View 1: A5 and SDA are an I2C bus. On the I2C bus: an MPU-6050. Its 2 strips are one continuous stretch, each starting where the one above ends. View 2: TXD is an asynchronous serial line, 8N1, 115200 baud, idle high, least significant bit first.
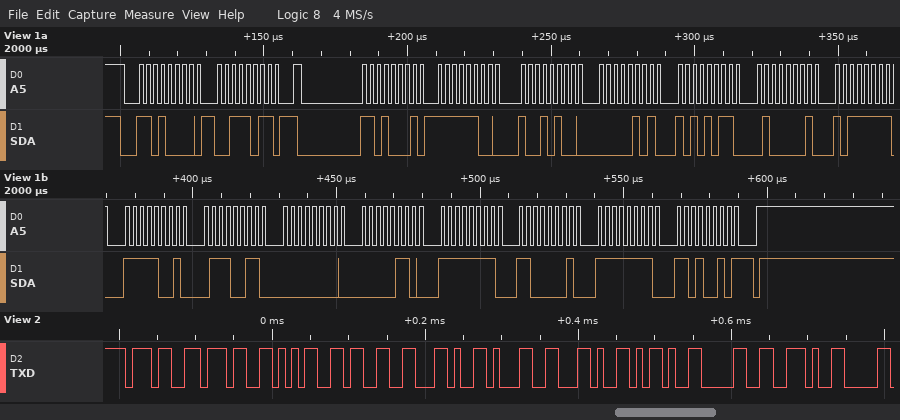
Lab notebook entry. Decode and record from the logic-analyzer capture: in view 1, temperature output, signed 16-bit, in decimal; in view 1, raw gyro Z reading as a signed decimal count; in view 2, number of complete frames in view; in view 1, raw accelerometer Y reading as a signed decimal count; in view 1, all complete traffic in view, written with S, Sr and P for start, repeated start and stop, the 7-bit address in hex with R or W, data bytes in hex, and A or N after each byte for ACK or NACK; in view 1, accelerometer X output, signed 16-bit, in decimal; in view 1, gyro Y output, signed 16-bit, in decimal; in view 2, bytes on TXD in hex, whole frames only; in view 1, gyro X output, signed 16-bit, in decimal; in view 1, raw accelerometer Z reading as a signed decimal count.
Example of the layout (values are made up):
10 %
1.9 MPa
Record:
-1677
-46
10
1451
S 68W A 3B A Sr 68R A FC A 94 A 05 A AB A 41 A BF A F9 A 73 A 00 A 06 A FF A C1 A FF A D2 N P
-876
-63
37 37 35 33 2C 31 2C 2D 30 2E
6
16831
